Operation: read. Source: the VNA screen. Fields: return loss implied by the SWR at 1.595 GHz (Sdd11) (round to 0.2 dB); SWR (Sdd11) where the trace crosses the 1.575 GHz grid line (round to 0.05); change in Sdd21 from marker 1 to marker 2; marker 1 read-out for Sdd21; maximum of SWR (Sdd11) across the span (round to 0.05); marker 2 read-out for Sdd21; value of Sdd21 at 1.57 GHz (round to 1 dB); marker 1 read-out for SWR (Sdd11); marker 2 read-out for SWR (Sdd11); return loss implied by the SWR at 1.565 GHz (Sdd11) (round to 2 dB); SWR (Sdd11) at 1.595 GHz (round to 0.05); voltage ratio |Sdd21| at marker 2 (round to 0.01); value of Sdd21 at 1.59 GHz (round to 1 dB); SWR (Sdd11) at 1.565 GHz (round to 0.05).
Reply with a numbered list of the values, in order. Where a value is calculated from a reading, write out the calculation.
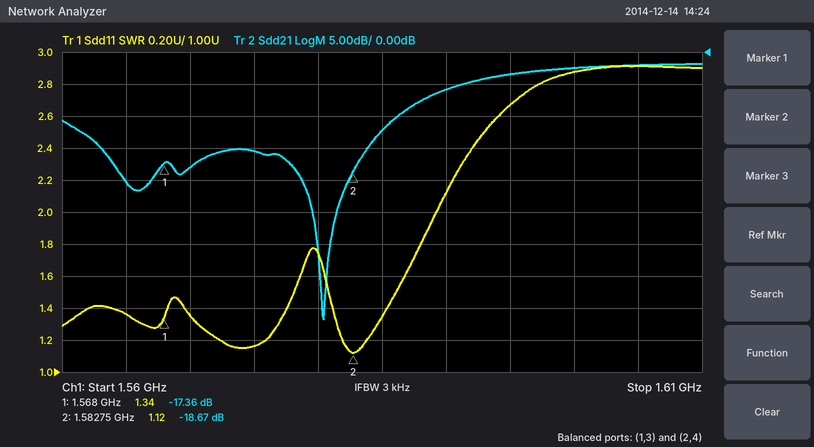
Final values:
1. −20 log10((2.65 − 1)/(2.65 + 1)) ≈ 6.90 dB, so 6.8 dB to the nearest 0.2 dB
2. 1.15
3. -18.67 − (-17.36) = -1.31 dB
4. -17.36 dB
5. 2.90
6. -18.67 dB
7. -18 dB
8. 1.34
9. 1.12
10. −20 log10((1.35 − 1)/(1.35 + 1)) ≈ 16 dB
11. 2.65
12. 10^(-18.67/20) ≈ 0.12
13. -6 dB
14. 1.35
